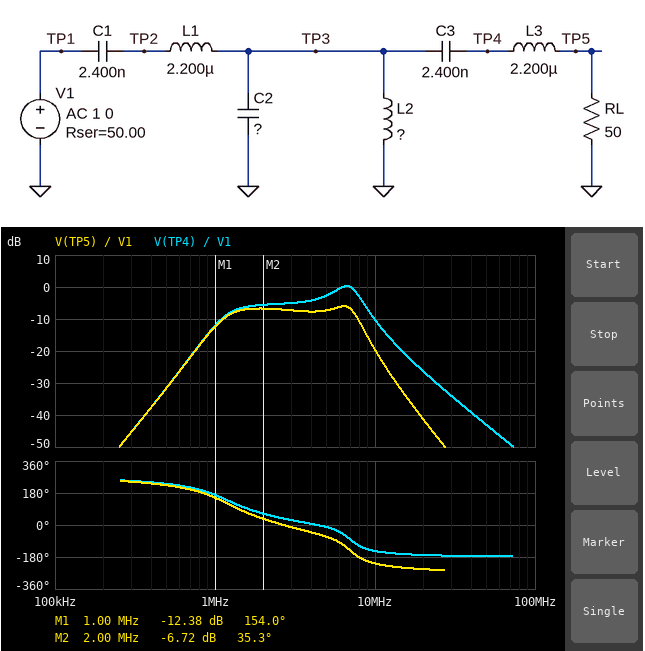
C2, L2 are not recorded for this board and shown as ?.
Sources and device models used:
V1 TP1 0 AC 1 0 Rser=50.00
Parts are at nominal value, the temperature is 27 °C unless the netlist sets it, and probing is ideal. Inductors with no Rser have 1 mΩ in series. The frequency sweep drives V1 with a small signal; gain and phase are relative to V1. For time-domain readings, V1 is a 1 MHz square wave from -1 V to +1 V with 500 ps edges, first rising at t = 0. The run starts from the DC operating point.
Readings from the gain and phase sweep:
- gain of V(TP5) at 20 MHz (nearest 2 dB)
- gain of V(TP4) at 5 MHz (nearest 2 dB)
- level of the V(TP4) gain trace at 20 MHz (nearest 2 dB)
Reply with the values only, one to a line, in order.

-42 dB
-2 dB
-26 dB
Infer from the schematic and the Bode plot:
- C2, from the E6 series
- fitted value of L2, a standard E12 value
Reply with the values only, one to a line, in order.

680 pF
2.7 µH
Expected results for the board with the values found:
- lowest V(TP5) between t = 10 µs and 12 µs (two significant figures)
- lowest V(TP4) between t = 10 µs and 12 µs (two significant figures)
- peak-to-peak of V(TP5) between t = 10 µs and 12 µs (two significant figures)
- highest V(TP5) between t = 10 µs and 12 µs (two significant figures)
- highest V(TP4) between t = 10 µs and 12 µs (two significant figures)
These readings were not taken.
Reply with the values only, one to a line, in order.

-410 mV
-620 mV
810 mV
410 mV
620 mV
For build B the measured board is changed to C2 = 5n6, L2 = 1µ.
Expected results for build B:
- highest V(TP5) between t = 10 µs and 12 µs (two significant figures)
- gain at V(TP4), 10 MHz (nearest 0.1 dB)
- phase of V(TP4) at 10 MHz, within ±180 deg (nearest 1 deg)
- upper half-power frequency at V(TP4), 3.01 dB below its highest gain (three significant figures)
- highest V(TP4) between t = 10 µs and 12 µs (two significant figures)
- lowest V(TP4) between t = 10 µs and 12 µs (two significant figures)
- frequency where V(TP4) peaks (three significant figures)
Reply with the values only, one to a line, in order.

240 mV
-32.8 dB
-157 deg
3.08 MHz
280 mV
-280 mV
2.19 MHz
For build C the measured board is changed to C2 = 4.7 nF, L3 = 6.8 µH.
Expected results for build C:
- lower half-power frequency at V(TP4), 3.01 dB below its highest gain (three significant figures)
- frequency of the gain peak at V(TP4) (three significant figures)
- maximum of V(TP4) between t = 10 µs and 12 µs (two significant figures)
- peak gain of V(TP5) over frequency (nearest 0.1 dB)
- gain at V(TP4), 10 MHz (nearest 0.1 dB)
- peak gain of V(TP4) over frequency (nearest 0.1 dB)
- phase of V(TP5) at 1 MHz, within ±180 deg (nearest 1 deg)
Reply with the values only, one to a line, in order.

1.00 MHz
1.66 MHz
860 mV
-6.1 dB
-31.8 dB
-1.7 dB
96 deg
